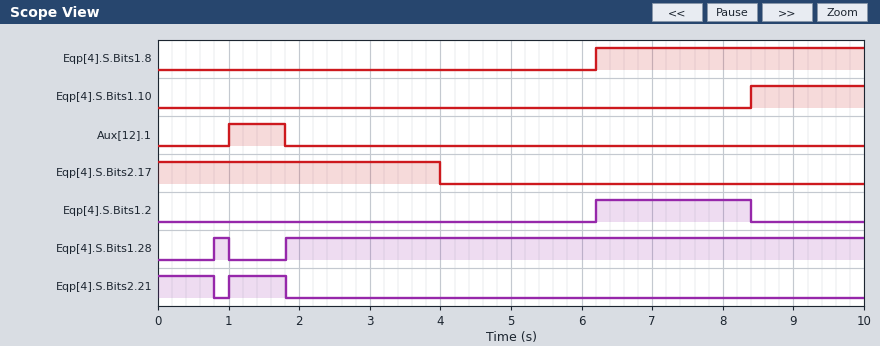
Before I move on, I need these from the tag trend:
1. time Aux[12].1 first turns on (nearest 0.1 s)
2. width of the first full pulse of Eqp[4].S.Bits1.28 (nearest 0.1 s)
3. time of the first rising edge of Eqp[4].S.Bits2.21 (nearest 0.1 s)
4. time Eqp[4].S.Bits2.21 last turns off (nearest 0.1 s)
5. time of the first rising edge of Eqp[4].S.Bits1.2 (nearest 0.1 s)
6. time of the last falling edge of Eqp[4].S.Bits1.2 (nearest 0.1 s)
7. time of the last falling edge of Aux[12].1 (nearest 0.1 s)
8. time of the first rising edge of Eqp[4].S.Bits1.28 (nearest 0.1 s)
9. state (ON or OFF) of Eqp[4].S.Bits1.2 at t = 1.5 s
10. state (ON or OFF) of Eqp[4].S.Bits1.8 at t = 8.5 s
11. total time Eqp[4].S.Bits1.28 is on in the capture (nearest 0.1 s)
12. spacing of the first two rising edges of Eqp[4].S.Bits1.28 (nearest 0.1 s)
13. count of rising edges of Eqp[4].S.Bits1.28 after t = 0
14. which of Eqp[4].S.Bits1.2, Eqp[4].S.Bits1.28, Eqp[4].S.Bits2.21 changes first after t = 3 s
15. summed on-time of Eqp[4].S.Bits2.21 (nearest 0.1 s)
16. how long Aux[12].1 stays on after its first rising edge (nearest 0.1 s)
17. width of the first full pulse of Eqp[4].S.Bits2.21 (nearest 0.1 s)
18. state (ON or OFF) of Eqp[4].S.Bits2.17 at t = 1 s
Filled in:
1.0 s
0.2 s
1.0 s
1.8 s
6.2 s
8.4 s
1.8 s
0.8 s
OFF
ON
8.4 s
1.0 s
2
Eqp[4].S.Bits1.2
1.6 s
0.8 s
0.8 s
ON
